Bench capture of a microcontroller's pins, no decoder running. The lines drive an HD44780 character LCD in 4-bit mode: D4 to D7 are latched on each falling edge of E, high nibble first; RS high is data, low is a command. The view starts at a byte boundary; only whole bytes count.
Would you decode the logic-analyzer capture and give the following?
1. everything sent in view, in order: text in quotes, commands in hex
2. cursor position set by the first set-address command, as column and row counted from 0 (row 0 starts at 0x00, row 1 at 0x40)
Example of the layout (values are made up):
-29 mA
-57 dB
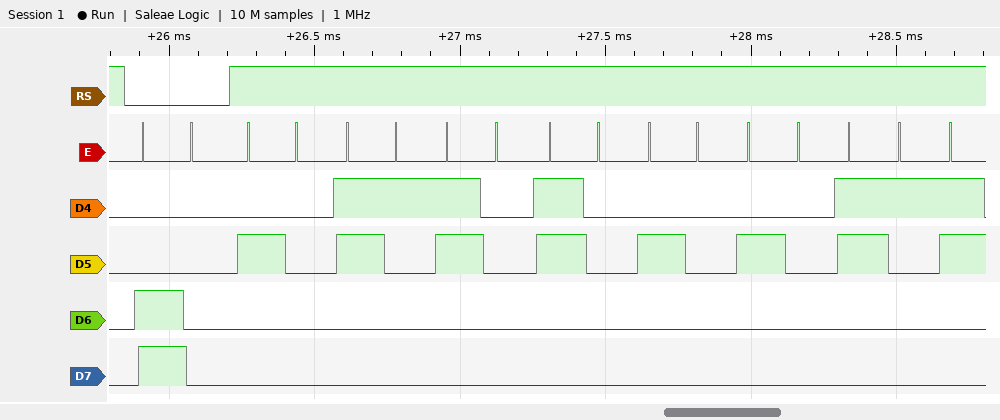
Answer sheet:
0xC0 " 100  1"
column 0, row 1
